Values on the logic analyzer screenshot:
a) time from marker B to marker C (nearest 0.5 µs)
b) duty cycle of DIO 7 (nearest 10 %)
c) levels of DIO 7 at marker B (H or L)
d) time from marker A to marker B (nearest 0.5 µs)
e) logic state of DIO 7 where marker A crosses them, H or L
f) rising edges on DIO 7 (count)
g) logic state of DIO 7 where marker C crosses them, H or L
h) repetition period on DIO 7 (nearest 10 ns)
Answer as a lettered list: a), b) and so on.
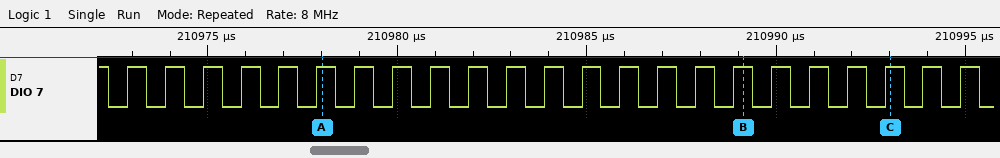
a) 4 µs
b) 50 %
c) DIO 7=H
d) 11 µs
e) DIO 7=H
f) 23
g) DIO 7=H
h) 1000 ns
